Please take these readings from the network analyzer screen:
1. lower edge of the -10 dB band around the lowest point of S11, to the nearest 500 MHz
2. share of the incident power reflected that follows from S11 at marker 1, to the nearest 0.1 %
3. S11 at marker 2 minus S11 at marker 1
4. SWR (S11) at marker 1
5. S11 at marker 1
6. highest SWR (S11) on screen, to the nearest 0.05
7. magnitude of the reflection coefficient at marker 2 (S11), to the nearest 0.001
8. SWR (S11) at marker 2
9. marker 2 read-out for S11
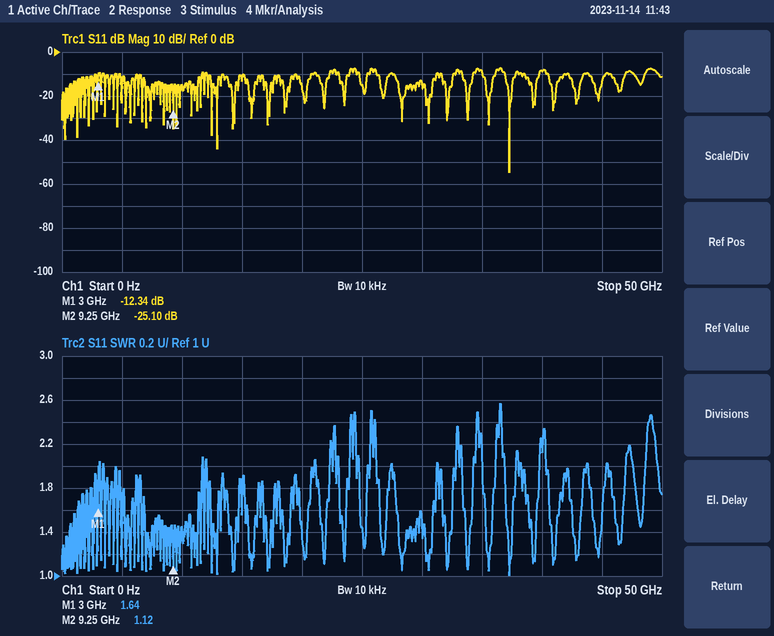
37.0 GHz
5.8 %
-12.76 dB
1.64
-12.34 dB
2.55
0.056
1.12
-25.10 dB
